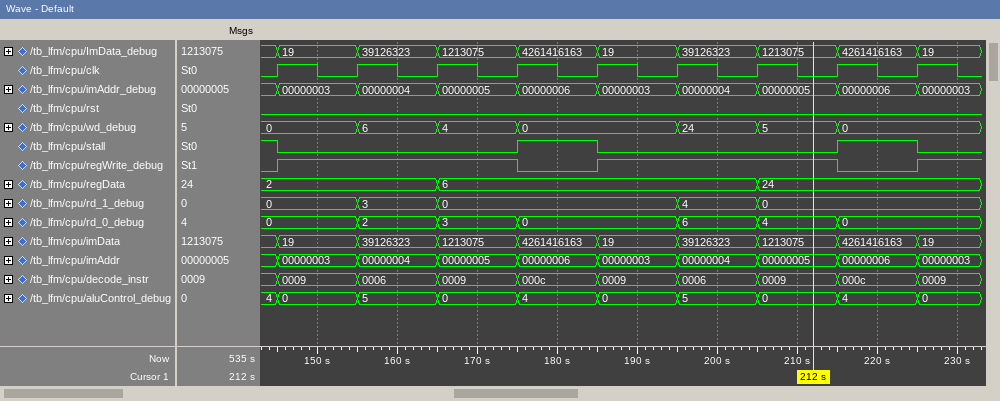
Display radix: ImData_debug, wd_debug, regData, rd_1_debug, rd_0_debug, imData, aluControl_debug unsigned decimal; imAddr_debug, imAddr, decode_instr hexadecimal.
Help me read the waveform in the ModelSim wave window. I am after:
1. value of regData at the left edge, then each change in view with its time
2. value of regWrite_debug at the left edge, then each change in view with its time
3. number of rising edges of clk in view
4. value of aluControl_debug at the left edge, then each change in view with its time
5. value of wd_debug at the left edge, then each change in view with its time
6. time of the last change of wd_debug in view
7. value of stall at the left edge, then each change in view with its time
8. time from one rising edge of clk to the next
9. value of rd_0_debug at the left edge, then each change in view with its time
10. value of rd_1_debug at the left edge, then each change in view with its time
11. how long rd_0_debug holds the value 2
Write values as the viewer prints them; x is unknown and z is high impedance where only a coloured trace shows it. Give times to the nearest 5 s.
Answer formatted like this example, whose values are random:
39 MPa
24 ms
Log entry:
2, 6 at 165 s, 24 at 205 s
0, 1 at 145 s, 0 at 175 s, 1 at 185 s, 0 at 215 s, 1 at 225 s
9
4, 0 at 145 s, 5 at 155 s, 0 at 165 s, 4 at 175 s, 0 at 185 s, 5 at 195 s, 0 at 205 s, 4 at 215 s, 0 at 225 s
0, 6 at 155 s, 4 at 165 s, 0 at 175 s, 24 at 195 s, 5 at 205 s, 0 at 215 s
215 s
1, 0 at 145 s, 1 at 175 s, 0 at 185 s, 1 at 215 s, 0 at 225 s
10 s
0, 2 at 155 s, 3 at 165 s, 0 at 175 s, 6 at 195 s, 4 at 205 s, 0 at 215 s
0, 3 at 155 s, 0 at 165 s, 4 at 195 s, 0 at 205 s
10 s
